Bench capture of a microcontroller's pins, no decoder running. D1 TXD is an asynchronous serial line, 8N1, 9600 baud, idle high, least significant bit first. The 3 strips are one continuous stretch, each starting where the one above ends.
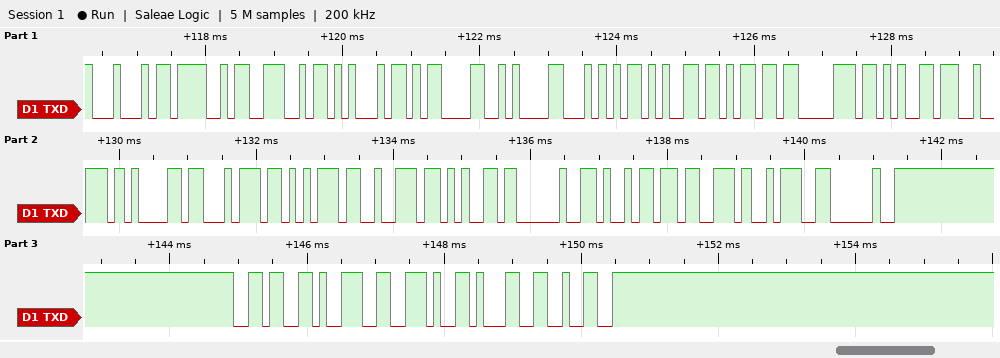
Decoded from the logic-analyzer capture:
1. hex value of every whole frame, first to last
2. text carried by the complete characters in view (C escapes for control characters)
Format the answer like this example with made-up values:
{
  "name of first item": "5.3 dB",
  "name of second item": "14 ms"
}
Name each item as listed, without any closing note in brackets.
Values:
{
  "hex value of every whole frame, first to last": "0x44 0x4F 0x4E 0x45 0x0D 0x0A 0x54 0x65 0x6D 0x70 0x65 0x72 0x61 0x74 0x75 0x72 0x65 0x20 0x69 0x73 0x3A 0x20 0x36 0x39 0x2E 0x31 0x32",
  "text carried by the complete characters in view": "\"DONE\\r\\nTemperature is: 69.12\""
}
